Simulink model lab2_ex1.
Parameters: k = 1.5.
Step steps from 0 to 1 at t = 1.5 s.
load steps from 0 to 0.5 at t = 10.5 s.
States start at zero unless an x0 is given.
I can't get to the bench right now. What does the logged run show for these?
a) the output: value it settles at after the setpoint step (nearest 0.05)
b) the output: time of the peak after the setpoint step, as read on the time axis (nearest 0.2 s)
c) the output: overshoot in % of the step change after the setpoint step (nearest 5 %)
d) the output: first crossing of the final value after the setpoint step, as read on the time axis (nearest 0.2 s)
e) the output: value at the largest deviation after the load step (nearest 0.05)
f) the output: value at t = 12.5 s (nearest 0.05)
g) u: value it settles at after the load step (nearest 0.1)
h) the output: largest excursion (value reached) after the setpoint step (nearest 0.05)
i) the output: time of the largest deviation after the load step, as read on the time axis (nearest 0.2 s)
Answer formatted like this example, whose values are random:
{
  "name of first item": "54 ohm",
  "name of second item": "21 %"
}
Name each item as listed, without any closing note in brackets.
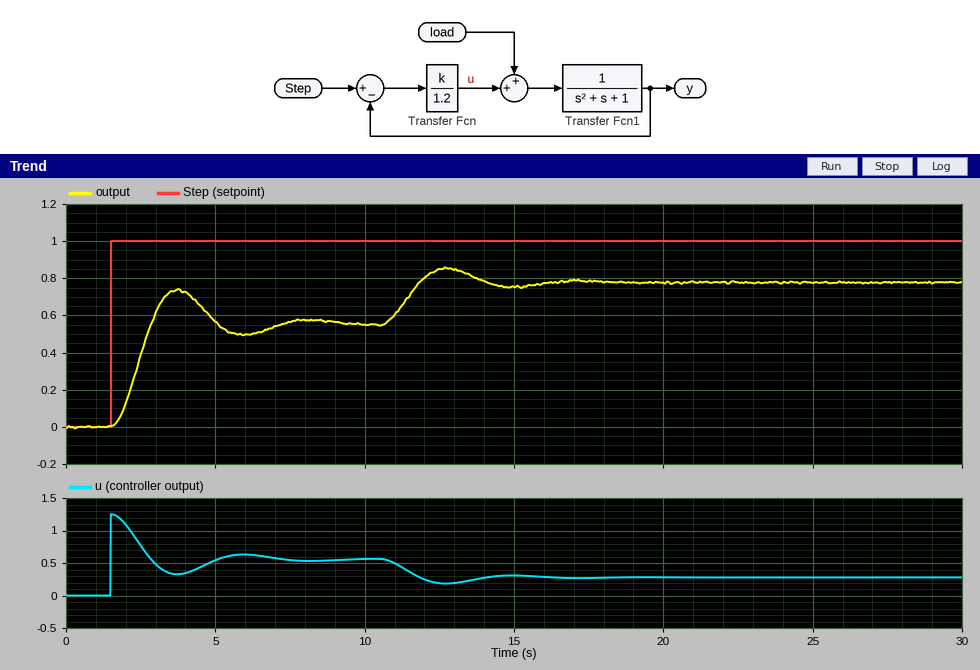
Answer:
{
  "the output: value it settles at after the setpoint step": "0.55",
  "the output: time of the peak after the setpoint step, as read on the time axis": "3.8 s",
  "the output: overshoot in % of the step change after the setpoint step": "35 %",
  "the output: first crossing of the final value after the setpoint step, as read on the time axis": "2.8 s",
  "the output: value at the largest deviation after the load step": "0.85",
  "the output: value at t = 12.5 s": "0.85",
  "u: value it settles at after the load step": "0.3",
  "the output: largest excursion (value reached) after the setpoint step": "0.75",
  "the output: time of the largest deviation after the load step, as read on the time axis": "12.8 s"
}
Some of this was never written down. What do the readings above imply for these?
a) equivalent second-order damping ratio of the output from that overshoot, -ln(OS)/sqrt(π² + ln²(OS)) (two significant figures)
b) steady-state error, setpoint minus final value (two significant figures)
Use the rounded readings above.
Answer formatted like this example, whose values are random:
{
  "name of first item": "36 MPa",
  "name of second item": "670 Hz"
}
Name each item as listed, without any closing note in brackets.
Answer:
{
  "equivalent second-order damping ratio of the output from that overshoot, -ln(OS)/sqrt(π² + ln²(OS))": "0.32",
  "steady-state error, setpoint minus final value": "0.45"
}
